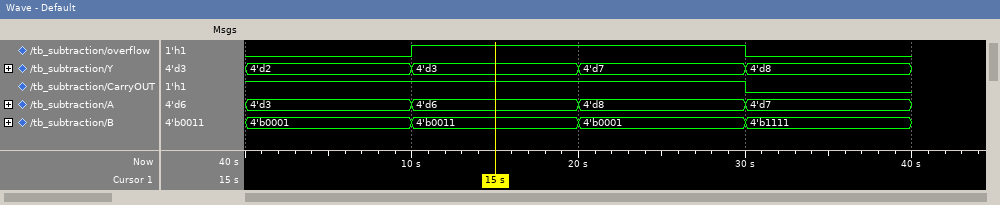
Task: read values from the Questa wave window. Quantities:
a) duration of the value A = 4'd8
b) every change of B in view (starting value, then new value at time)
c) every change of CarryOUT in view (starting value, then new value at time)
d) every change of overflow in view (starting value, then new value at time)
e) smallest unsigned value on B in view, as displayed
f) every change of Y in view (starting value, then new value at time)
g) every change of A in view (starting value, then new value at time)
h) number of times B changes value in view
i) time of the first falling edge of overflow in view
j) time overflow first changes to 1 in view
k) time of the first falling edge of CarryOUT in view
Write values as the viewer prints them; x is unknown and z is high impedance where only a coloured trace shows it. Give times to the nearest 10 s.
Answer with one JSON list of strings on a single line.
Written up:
["10 s", "4'b0001, 4'b0011 at 10 s, 4'b0001 at 20 s, 4'b1111 at 30 s", "1, 0 at 30 s", "0, 1 at 10 s, 0 at 30 s", "4'b0001", "4'd2, 4'd3 at 10 s, 4'd7 at 20 s, 4'd8 at 30 s", "4'd3, 4'd6 at 10 s, 4'd8 at 20 s, 4'd7 at 30 s", "3", "30 s", "10 s", "30 s"]
